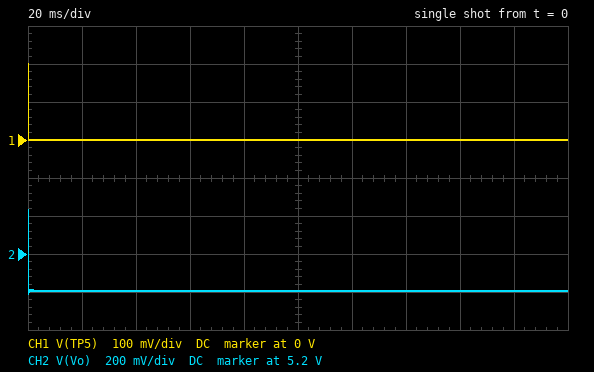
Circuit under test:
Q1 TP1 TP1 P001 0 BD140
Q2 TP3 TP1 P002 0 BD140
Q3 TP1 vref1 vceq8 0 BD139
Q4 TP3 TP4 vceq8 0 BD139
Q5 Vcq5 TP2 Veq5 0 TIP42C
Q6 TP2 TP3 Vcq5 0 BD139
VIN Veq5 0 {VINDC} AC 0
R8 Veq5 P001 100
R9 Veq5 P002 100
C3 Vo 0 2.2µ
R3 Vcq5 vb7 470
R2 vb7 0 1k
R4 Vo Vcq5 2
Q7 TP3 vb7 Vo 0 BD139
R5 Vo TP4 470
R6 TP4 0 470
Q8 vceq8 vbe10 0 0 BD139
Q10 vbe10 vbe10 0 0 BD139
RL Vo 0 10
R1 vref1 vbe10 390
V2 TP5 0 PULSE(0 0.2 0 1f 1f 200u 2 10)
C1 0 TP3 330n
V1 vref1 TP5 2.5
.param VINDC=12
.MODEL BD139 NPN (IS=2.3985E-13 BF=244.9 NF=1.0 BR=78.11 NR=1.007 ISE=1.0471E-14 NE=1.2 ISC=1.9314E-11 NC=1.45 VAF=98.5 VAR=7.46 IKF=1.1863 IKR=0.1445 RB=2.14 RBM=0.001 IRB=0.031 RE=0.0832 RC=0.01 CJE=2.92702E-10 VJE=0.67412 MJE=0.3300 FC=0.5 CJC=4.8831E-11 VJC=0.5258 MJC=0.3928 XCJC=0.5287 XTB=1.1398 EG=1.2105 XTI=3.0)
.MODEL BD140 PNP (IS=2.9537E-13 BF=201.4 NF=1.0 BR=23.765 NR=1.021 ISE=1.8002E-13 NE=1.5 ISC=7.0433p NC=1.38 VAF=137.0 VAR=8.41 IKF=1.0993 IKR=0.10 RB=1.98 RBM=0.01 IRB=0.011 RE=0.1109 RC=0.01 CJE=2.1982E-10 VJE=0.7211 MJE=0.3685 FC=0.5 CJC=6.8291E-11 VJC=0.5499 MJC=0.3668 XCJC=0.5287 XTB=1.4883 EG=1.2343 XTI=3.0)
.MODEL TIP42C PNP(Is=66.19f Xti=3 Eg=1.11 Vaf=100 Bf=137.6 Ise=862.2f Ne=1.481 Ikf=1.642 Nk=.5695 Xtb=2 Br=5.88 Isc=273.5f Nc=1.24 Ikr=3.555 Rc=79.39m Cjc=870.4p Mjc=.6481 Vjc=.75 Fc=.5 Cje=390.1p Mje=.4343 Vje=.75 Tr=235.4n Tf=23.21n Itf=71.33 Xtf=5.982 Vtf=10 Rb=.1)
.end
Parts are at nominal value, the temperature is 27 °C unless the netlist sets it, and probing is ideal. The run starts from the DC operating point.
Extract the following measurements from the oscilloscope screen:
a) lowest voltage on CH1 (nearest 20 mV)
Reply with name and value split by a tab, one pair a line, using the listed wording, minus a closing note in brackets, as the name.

lowest voltage on CH1	0 V
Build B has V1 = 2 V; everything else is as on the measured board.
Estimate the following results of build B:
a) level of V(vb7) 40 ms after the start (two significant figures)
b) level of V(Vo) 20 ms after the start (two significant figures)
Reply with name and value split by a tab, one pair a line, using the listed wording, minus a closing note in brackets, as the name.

level of V(vb7) 40 ms after the start	3.3 V
level of V(Vo) 20 ms after the start	4.0 V
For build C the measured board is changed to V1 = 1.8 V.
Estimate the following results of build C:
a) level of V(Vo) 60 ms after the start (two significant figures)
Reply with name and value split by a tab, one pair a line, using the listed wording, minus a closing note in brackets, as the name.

level of V(Vo) 60 ms after the start	3.6 V
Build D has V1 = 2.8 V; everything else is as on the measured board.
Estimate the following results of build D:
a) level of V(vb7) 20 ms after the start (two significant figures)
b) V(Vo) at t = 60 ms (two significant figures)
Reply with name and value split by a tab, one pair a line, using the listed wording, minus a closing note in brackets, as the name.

level of V(vb7) 20 ms after the start	4.6 V
V(Vo) at t = 60 ms	5.6 V
